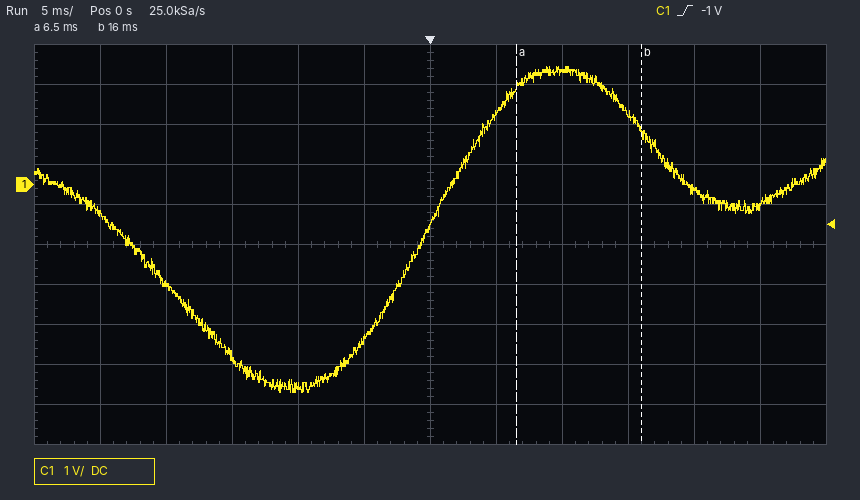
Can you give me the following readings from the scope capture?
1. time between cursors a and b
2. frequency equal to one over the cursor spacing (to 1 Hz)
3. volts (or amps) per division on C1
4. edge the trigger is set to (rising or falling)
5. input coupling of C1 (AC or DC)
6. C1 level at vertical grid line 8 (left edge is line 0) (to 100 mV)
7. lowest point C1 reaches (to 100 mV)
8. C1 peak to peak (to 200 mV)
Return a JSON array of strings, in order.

["9.5 ms", "105 Hz", "1 V", "rising", "DC", "2.8 V", "-5.2 V", "8.2 V"]
